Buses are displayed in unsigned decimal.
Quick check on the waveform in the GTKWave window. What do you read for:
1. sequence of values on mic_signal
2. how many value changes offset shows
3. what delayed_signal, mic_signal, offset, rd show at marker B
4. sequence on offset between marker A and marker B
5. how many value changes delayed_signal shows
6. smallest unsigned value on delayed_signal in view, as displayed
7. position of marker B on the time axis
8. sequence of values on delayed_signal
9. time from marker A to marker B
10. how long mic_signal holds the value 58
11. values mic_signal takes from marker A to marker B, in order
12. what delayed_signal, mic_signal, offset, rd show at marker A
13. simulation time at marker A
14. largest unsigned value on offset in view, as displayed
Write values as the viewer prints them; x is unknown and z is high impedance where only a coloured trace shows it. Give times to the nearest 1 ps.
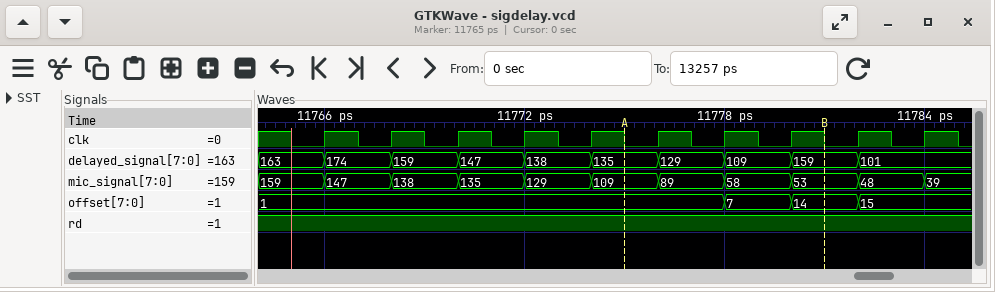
159, 147, 138, 135, 129, 109, 89, 58, 53, 48, 39
3
delayed_signal=159, mic_signal=53, offset=14, rd=1
1, 7, 14
9
101
11781 ps
163, 174, 159, 147, 138, 135, 129, 109, 159, 101
6 ps
2 ps
109, 89, 58, 53
delayed_signal=135, mic_signal=109, offset=1, rd=1
11775 ps
15
